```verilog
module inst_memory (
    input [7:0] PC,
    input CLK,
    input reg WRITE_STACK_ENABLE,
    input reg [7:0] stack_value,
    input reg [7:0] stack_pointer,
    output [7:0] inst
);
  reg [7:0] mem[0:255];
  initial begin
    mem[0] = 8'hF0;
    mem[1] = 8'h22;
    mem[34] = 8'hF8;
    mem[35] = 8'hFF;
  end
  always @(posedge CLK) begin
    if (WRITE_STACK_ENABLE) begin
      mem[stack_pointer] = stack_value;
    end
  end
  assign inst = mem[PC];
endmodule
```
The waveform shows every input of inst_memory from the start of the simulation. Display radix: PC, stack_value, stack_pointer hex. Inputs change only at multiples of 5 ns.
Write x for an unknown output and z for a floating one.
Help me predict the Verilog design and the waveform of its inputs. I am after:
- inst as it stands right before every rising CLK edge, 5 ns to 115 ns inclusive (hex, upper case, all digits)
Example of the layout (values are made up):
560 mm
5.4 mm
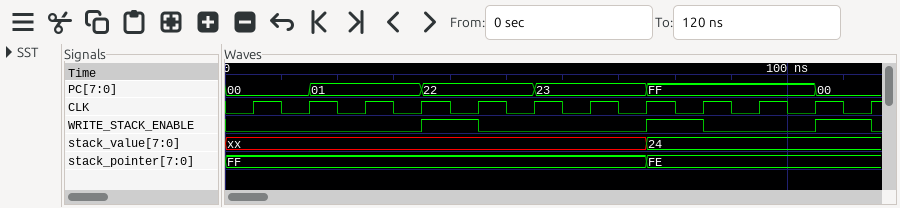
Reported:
F0, F0, 22, 22, F8, F8, FF, FF, x, x, x, F0
